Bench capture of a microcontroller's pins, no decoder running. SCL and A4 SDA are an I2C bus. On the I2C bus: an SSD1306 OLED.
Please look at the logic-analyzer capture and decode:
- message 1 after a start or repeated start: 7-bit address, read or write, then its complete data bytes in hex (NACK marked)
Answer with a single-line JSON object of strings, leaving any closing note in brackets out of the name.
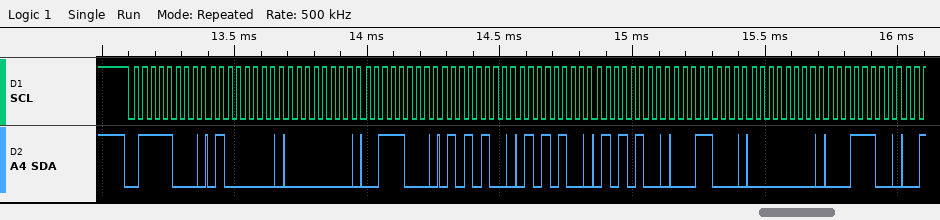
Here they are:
{"message 1 after a start or repeated start: 7-bit address, read or write, then its complete data bytes in hex": "0x3C write: 40 00 38 54 54 54 18 00 1C"}
